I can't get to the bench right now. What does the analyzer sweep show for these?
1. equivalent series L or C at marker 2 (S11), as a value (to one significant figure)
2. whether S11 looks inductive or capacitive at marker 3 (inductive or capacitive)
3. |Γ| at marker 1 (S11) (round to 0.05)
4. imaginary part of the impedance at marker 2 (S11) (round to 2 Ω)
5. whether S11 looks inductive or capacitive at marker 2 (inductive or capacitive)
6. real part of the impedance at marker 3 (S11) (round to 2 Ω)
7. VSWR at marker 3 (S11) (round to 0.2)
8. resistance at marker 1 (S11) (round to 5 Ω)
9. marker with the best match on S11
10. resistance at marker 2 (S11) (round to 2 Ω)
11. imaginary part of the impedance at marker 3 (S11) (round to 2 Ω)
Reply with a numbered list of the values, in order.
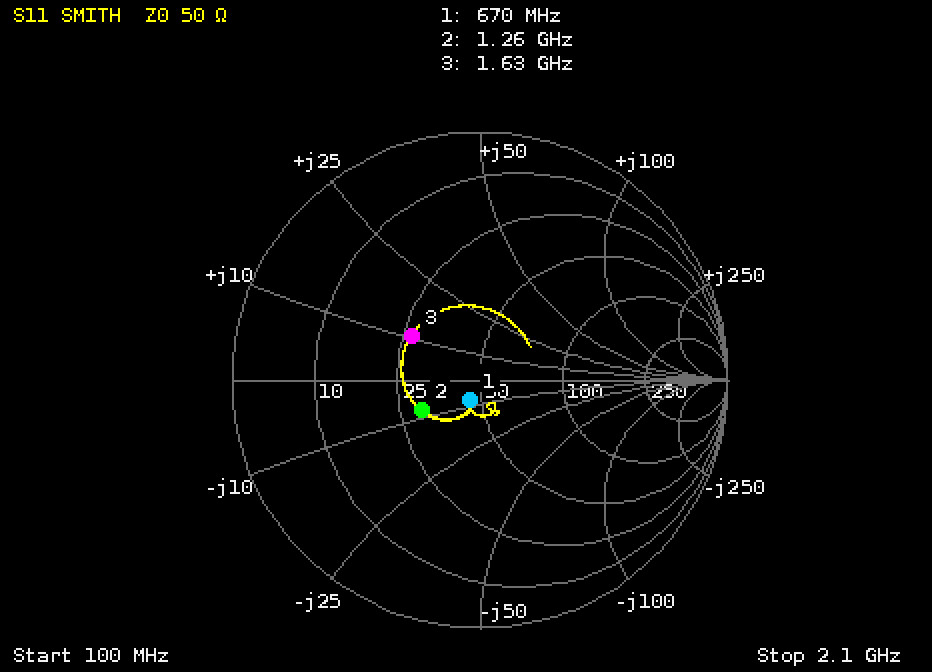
1. 20 pF
2. inductive
3. 0.10
4. -8 Ω
5. capacitive
6. 26 Ω
7. 2.0
8. 45 Ω
9. marker 1
10. 30 Ω
11. +10 Ω
